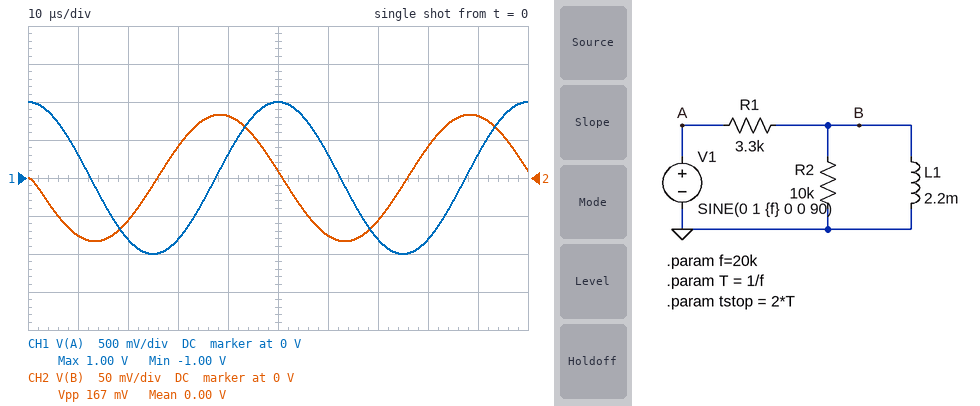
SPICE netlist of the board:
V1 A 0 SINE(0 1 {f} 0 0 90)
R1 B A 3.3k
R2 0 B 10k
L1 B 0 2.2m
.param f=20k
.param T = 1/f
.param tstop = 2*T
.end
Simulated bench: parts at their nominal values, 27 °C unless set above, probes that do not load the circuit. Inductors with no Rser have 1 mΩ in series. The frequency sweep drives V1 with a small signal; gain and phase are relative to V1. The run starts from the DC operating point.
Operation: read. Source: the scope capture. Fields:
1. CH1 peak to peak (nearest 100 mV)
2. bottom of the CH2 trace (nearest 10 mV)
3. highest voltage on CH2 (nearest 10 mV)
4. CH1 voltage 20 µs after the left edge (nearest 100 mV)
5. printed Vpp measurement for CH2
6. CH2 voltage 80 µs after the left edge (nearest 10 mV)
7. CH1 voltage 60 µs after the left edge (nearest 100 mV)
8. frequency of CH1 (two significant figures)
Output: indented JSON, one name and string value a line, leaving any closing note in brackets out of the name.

{
  "CH1 peak to peak": "2.0 V",
  "bottom of the CH2 trace": "-80 mV",
  "highest voltage on CH2": "80 mV",
  "CH1 voltage 20 µs after the left edge": "-800 mV",
  "printed Vpp measurement for CH2": "167 mV",
  "CH2 voltage 80 µs after the left edge": "40 mV",
  "CH1 voltage 60 µs after the left edge": "300 mV",
  "frequency of CH1": "20 kHz"
}
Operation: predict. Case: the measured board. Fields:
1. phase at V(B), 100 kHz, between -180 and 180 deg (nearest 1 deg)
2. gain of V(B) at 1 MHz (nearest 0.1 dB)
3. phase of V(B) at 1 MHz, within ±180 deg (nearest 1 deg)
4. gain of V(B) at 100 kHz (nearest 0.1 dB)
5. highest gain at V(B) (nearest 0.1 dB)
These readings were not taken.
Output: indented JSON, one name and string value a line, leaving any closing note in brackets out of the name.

{
  "phase at V(B), 100 kHz, between -180 and 180 deg": "61 deg",
  "gain of V(B) at 1 MHz": "-2.6 dB",
  "phase of V(B) at 1 MHz, within ±180 deg": "10 deg",
  "gain of V(B) at 100 kHz": "-8.7 dB",
  "highest gain at V(B)": "-2.5 dB"
}
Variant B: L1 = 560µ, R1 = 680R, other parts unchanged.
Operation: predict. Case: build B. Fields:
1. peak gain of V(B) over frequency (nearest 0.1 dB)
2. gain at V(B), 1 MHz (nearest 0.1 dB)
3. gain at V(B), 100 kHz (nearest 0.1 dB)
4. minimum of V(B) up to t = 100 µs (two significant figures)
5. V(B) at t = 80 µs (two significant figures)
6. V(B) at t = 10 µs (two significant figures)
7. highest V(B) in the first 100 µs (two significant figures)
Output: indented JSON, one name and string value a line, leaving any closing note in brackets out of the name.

{
  "peak gain of V(B) over frequency": "-0.6 dB",
  "gain at V(B), 1 MHz": "-0.7 dB",
  "gain at V(B), 100 kHz": "-6.9 dB",
  "minimum of V(B) up to t = 100 µs": "-100 mV",
  "V(B) at t = 80 µs": "51 mV",
  "V(B) at t = 10 µs": "-94 mV",
  "highest V(B) in the first 100 µs": "100 mV"
}
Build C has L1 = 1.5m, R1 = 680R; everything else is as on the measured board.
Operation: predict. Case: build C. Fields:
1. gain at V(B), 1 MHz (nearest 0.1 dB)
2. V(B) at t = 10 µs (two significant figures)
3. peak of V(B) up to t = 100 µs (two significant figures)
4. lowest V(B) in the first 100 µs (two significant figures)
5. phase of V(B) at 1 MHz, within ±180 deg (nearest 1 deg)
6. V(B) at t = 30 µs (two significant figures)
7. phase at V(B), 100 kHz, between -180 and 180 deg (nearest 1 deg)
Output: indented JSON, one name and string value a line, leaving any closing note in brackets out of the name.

{
  "gain at V(B), 1 MHz": "-0.6 dB",
  "V(B) at t = 10 µs": "-220 mV",
  "peak of V(B) up to t = 100 µs": "270 mV",
  "lowest V(B) in the first 100 µs": "-270 mV",
  "phase of V(B) at 1 MHz, within ±180 deg": "4 deg",
  "V(B) at t = 30 µs": "89 mV",
  "phase at V(B), 100 kHz, between -180 and 180 deg": "34 deg"
}
